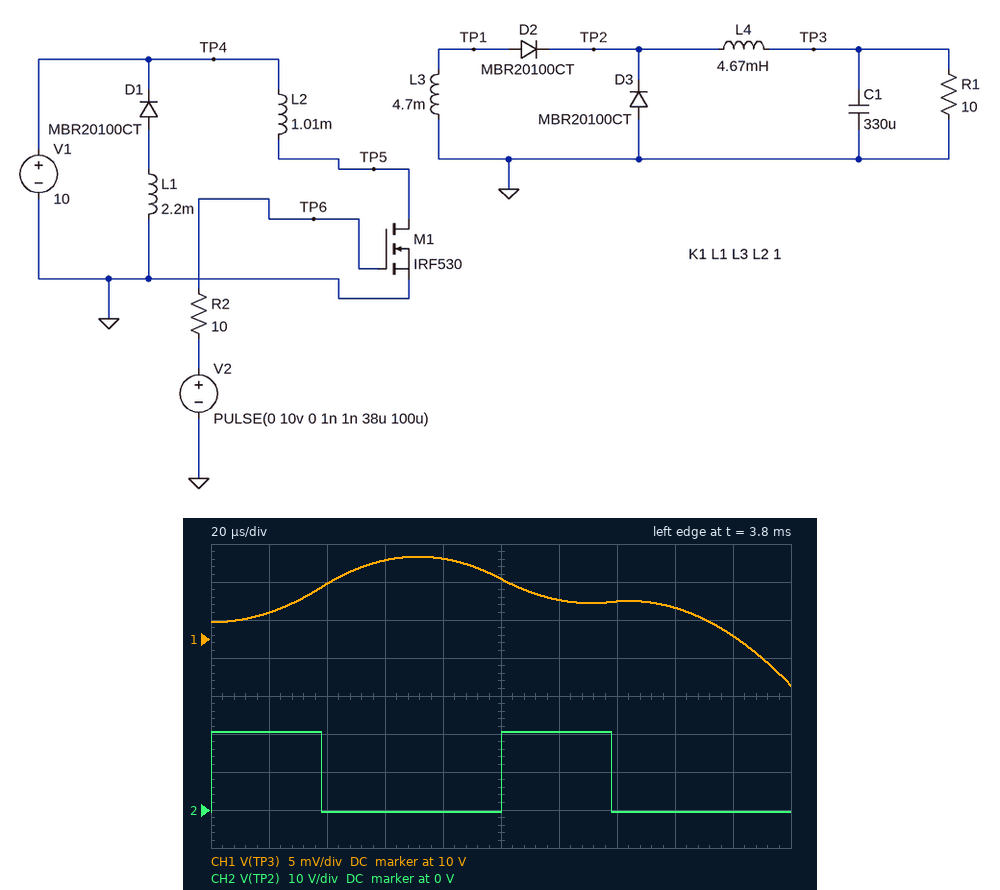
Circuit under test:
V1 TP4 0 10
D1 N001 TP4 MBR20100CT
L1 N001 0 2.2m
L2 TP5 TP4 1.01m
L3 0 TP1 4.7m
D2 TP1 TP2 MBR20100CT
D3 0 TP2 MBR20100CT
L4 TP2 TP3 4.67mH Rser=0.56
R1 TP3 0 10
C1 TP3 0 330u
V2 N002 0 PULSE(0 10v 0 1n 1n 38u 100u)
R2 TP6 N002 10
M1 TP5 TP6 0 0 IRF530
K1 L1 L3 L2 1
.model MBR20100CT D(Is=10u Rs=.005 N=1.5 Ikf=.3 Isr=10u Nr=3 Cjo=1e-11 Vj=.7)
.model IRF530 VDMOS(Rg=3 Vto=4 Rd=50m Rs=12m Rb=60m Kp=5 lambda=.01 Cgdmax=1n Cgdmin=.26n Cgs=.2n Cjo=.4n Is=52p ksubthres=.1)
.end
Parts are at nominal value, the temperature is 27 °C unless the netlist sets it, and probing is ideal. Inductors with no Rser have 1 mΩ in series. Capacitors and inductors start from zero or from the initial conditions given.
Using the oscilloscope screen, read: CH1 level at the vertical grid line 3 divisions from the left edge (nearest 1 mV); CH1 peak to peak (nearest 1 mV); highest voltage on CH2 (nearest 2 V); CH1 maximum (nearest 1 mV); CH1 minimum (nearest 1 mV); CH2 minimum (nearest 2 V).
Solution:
10.010 V
17 mV
20 V
10.011 V
9.994 V
0 V
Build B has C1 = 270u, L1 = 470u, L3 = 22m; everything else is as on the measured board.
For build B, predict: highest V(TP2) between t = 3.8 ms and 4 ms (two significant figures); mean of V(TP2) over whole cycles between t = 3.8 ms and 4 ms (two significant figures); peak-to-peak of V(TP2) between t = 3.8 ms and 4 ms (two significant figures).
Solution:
43 V
16 V
44 V
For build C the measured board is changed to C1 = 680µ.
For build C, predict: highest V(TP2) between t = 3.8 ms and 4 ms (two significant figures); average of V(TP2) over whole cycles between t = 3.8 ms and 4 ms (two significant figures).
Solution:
20 V
7.2 V
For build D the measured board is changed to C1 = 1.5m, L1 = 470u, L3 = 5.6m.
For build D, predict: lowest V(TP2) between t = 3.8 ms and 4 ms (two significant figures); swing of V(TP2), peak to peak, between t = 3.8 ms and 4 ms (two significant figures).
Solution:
-620 mV
22 V
